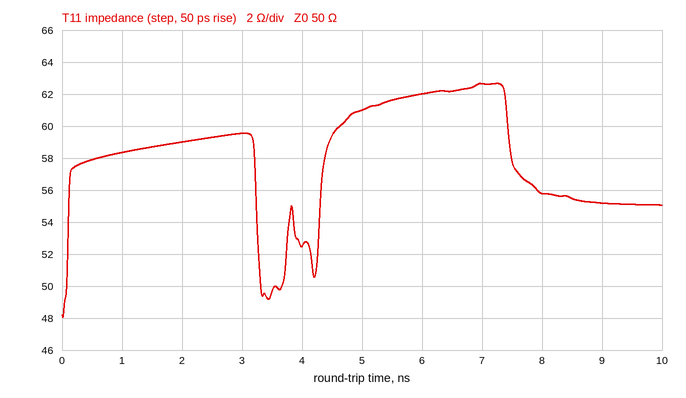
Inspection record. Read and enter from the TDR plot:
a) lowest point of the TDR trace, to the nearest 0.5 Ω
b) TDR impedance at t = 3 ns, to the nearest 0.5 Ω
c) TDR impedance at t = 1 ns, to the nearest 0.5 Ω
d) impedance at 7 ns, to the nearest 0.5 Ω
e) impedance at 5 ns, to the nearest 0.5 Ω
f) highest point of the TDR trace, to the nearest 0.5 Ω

48.0 Ω
59.5 Ω
58.5 Ω
62.5 Ω
61.0 Ω
62.5 Ω
